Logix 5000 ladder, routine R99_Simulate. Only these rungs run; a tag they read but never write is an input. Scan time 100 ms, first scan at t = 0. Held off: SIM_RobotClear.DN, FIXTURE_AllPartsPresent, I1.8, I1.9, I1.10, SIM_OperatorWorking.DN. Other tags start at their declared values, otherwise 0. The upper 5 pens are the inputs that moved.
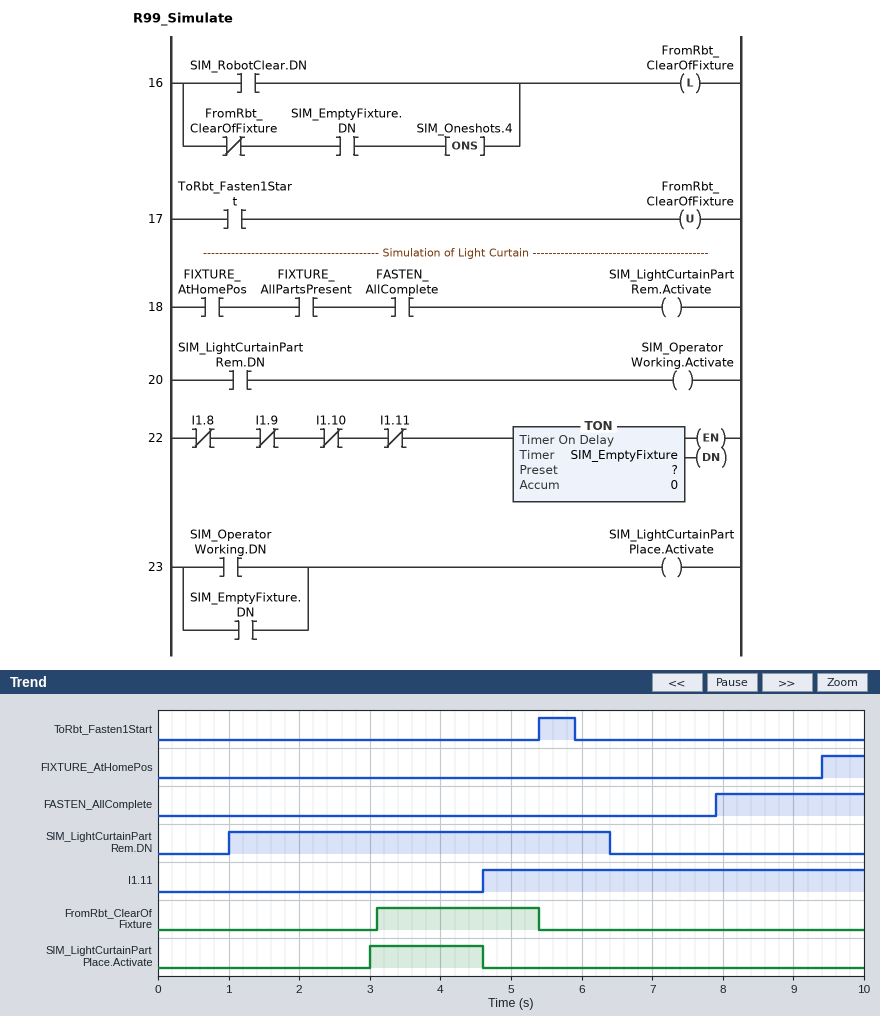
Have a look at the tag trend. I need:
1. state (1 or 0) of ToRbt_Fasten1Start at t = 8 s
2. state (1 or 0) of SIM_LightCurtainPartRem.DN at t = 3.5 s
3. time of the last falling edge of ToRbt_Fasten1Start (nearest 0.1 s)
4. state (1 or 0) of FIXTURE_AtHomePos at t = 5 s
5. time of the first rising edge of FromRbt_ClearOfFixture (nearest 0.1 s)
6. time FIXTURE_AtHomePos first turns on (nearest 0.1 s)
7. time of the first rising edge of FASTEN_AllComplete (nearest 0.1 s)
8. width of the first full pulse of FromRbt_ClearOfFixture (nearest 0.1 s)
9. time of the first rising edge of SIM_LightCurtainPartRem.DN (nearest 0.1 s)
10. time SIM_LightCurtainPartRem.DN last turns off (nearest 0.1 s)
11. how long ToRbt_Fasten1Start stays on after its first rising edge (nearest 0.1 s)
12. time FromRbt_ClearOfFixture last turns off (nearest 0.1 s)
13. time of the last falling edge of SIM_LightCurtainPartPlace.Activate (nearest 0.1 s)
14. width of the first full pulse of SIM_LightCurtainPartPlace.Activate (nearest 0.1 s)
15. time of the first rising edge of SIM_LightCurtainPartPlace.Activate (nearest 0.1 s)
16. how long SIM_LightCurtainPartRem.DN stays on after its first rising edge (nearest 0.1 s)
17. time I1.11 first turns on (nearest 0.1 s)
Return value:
0
1
5.9 s
0
3.1 s
9.4 s
7.9 s
2.3 s
1.0 s
6.4 s
0.5 s
5.4 s
4.6 s
1.6 s
3.0 s
5.4 s
4.6 s
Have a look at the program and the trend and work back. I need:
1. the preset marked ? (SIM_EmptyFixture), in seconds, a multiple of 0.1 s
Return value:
3.0 s
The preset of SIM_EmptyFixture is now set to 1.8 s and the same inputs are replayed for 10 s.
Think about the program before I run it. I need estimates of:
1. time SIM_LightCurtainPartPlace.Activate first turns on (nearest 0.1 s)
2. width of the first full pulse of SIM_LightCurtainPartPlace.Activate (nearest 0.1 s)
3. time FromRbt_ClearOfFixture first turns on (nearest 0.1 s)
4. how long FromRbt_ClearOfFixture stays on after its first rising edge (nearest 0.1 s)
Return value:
1.8 s
2.8 s
1.9 s
3.5 s
